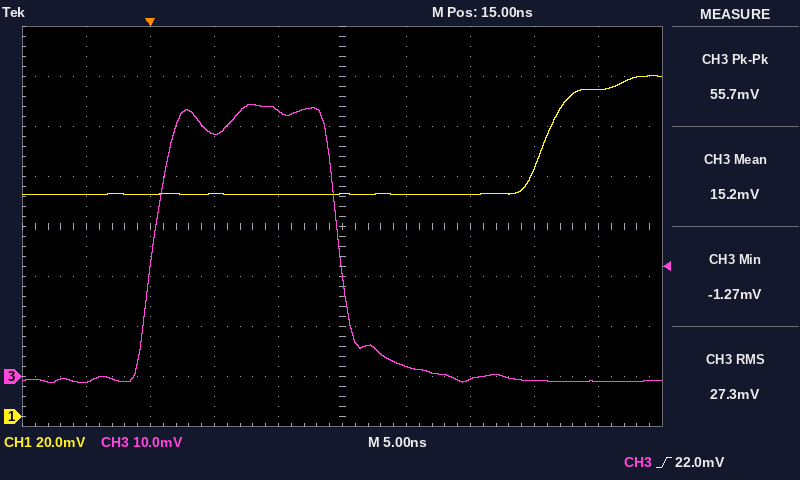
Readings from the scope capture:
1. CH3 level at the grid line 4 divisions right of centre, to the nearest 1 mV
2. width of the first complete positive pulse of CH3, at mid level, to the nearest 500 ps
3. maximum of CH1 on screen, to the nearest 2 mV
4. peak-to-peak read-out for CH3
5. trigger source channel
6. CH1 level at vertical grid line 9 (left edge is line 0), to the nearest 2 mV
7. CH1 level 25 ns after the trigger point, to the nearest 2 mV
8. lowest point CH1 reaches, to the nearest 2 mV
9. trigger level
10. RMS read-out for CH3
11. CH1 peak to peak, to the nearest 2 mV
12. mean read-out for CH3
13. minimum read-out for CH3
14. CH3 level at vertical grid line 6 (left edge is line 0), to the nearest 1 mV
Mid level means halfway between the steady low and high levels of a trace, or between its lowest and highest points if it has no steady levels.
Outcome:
-1 mV
14.5 ns
136 mV
55.7 mV
CH3
130 mV
88 mV
88 mV
22.0 mV
27.3 mV
48 mV
15.2 mV
-1.27 mV
2 mV
